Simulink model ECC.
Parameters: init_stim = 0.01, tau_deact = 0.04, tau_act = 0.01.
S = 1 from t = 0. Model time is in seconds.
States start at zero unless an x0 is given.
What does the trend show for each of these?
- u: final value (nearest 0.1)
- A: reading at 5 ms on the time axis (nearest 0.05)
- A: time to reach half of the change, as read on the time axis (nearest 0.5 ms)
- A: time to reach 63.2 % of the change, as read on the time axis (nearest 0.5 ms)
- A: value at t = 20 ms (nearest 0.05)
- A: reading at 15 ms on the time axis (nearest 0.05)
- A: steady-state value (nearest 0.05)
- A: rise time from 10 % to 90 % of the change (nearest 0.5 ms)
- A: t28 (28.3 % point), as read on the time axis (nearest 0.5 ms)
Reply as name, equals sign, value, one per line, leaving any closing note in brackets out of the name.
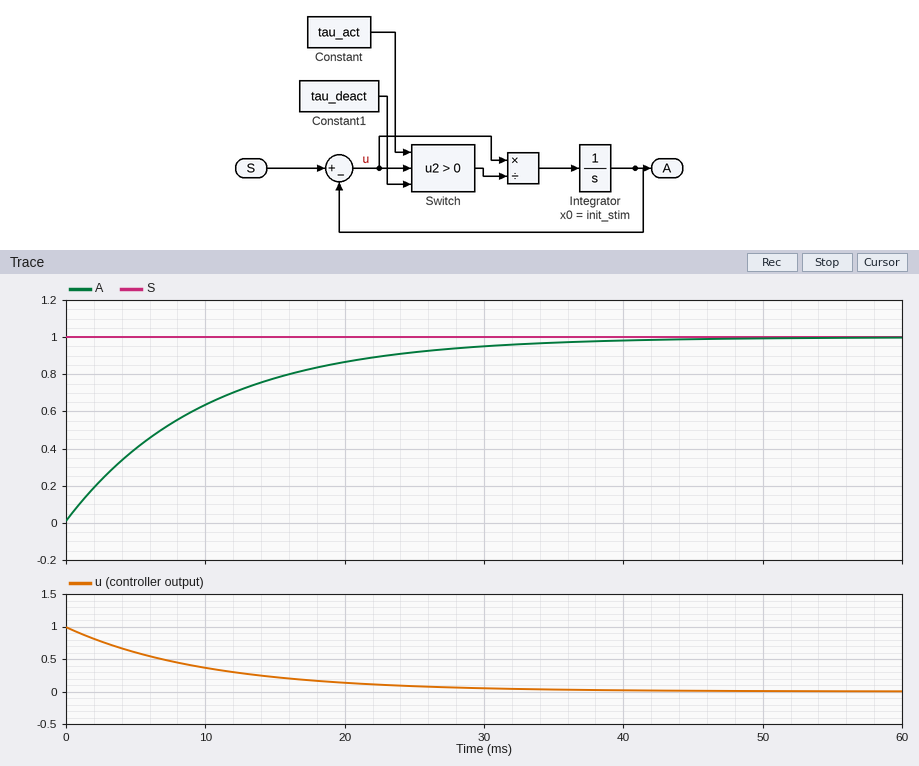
u: final value = 0.0
A: reading at 5 ms on the time axis = 0.40
A: time to reach half of the change, as read on the time axis = 7.0 ms
A: time to reach 63.2 % of the change, as read on the time axis = 10.0 ms
A: value at t = 20 ms = 0.85
A: reading at 15 ms on the time axis = 0.80
A: steady-state value = 1.00
A: rise time from 10 % to 90 % of the change = 22.0 ms
A: t28 (28.3 % point), as read on the time axis = 3.5 ms
